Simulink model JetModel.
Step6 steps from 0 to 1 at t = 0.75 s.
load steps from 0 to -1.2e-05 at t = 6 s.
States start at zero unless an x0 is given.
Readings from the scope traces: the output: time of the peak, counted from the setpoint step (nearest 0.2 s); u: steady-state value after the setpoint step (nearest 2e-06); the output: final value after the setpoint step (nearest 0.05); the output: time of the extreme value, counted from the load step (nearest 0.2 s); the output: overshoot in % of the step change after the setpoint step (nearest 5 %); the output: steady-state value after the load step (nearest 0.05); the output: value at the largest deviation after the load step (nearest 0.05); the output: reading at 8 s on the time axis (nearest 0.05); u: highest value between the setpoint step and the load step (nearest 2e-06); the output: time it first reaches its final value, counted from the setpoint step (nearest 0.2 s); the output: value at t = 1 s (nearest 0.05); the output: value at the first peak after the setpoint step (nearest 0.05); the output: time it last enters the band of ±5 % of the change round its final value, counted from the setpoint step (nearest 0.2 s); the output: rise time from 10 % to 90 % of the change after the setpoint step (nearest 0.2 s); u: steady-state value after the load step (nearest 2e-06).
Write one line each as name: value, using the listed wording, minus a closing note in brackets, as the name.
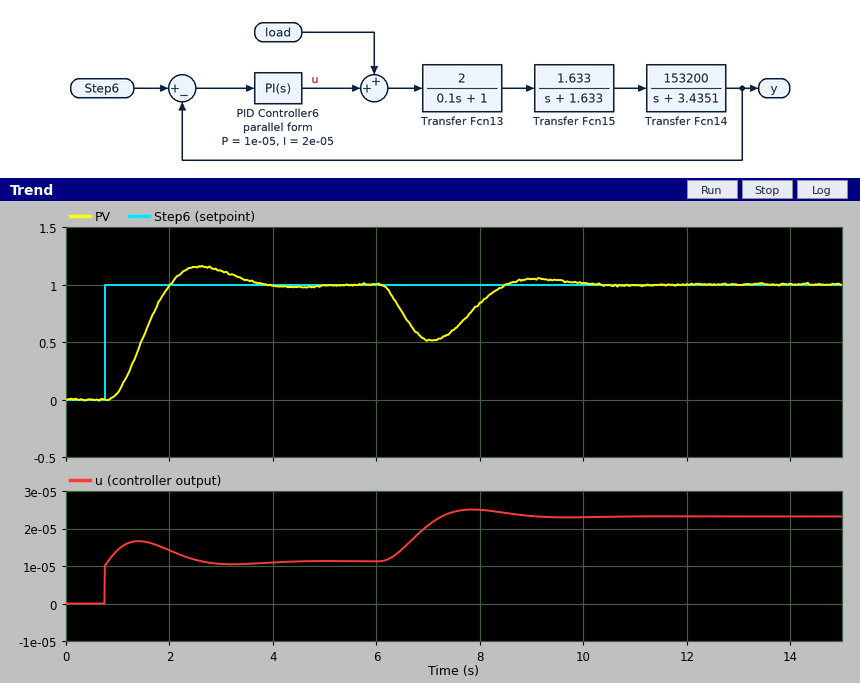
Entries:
the output: time of the peak, counted from the setpoint step: 1.8 s
u: steady-state value after the setpoint step: 0.000012
the output: final value after the setpoint step: 1.00
the output: time of the extreme value, counted from the load step: 1.0 s
the output: overshoot in % of the step change after the setpoint step: 15 %
the output: steady-state value after the load step: 1.00
the output: value at the largest deviation after the load step: 0.50
the output: reading at 8 s on the time axis: 0.85
u: highest value between the setpoint step and the load step: 0.000016
the output: time it first reaches its final value, counted from the setpoint step: 1.2 s
the output: value at t = 1 s: 0.05
the output: value at the first peak after the setpoint step: 1.15
the output: time it last enters the band of ±5 % of the change round its final value, counted from the setpoint step: 2.6 s
the output: rise time from 10 % to 90 % of the change after the setpoint step: 0.8 s
u: steady-state value after the load step: 0.000024
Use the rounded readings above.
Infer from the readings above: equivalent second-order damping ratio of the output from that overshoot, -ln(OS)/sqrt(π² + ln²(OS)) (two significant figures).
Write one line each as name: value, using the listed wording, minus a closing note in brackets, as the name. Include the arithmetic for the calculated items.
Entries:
equivalent second-order damping ratio of the output from that overshoot, -ln(OS)/sqrt(π² + ln²(OS)): ln(0.15) = -1.897; 1.897 / sqrt(9.870 + 3.599) = 0.52
